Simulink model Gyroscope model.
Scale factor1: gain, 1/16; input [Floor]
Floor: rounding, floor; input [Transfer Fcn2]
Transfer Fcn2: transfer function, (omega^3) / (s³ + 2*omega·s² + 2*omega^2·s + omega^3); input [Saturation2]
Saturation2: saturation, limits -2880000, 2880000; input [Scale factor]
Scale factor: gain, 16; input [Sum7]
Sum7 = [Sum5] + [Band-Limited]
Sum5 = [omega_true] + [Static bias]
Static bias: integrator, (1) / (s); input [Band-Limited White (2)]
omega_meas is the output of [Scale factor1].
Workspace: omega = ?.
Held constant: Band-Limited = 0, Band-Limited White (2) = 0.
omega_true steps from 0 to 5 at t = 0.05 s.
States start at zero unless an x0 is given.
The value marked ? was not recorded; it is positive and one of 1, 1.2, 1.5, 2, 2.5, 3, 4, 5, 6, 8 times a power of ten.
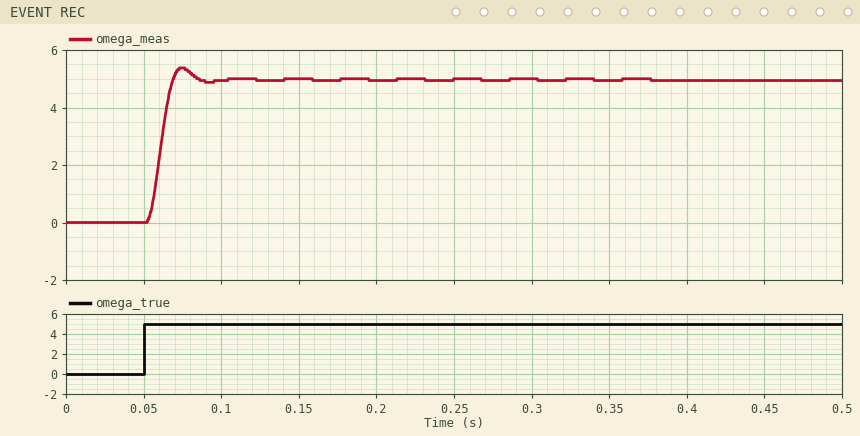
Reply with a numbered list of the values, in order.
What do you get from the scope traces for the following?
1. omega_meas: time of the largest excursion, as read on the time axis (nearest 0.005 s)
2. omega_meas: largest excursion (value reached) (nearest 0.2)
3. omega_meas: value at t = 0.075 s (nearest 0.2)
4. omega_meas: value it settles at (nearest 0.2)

1. 0.075 s
2. 5.4
3. 5.4
4. 5.0
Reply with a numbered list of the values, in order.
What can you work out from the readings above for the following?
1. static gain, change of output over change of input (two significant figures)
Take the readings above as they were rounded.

1. 1.0
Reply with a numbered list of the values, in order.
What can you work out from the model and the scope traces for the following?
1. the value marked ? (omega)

1. 200
